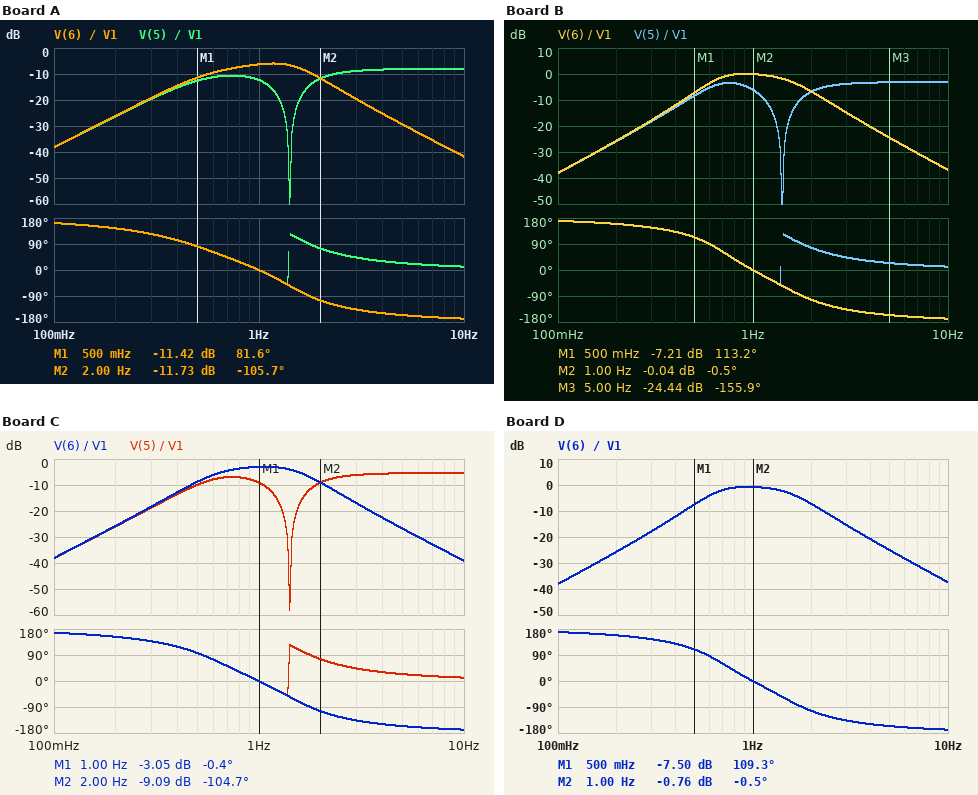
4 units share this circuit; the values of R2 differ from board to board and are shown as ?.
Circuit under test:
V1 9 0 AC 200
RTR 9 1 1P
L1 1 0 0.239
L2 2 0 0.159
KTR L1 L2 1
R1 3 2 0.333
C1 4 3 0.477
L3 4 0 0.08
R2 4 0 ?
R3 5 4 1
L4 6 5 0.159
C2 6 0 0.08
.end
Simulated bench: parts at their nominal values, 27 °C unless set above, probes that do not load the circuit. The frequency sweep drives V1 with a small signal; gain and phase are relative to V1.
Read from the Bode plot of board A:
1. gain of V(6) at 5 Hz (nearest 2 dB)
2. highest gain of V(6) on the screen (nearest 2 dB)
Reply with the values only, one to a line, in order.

-30 dB
-6 dB
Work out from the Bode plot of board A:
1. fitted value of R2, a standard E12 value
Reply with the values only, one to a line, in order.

0.33 Ω
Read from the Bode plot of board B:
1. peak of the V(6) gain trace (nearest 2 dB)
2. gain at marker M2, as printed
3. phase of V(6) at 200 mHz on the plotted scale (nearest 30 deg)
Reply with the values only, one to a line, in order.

0 dB
-0.04 dB
150 deg
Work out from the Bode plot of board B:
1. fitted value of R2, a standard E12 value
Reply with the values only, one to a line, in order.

2.2 Ω
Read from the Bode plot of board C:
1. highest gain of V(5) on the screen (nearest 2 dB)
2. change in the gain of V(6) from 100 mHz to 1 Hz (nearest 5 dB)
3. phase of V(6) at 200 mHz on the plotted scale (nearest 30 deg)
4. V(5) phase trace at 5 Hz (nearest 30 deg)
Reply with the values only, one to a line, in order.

-6 dB
35 dB
150 deg
30 deg
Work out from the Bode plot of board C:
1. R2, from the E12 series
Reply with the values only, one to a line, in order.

0.68 Ω
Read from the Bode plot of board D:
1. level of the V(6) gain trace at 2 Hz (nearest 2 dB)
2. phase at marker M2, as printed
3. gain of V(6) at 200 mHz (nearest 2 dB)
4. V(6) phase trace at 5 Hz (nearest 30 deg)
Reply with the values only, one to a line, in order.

-8 dB
-0.5 deg
-26 dB
-150 deg
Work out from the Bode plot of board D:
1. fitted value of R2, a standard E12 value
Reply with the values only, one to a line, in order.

1.5 Ω
